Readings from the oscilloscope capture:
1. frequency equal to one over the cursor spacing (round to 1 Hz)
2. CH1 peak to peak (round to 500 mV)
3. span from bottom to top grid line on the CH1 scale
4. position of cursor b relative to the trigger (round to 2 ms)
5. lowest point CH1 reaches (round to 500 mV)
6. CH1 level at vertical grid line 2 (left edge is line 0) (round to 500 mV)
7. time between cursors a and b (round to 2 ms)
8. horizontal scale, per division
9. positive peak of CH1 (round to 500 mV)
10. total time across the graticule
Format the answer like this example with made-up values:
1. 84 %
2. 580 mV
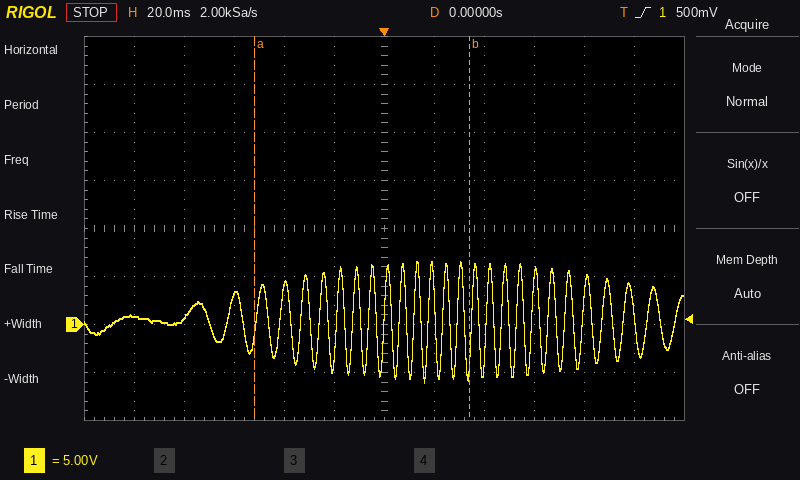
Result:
1. 12 Hz
2. 12.5 V
3. 40 V
4. +34 ms
5. -6.0 V
6. 500 mV
7. 86 ms
8. 20 ms
9. 6.5 V
10. 240 ms
